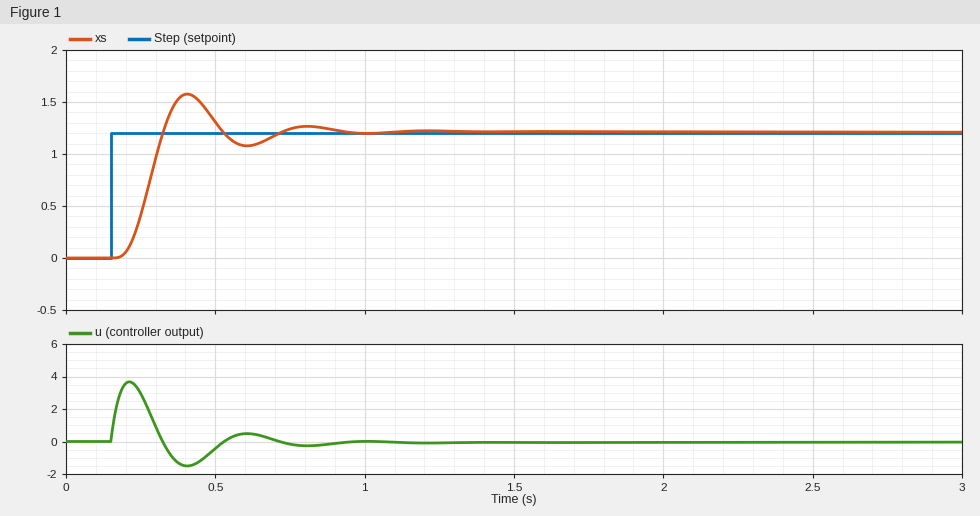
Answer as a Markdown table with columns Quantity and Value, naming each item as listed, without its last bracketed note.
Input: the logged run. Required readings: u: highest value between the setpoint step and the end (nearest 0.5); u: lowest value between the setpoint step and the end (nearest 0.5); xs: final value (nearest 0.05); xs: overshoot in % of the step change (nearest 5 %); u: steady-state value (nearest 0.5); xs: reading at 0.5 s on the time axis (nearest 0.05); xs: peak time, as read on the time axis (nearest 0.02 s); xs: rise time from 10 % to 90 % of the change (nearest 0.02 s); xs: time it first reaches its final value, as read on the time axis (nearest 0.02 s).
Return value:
| Quantity | Value |
|---|---|
| u: highest value between the setpoint step and the end | 3.5 |
| u: lowest value between the setpoint step and the end | -1.5 |
| xs: final value | 1.20 |
| xs: overshoot in % of the step change | 30 % |
| u: steady-state value | 0.0 |
| xs: reading at 0.5 s on the time axis | 1.30 |
| xs: peak time, as read on the time axis | 0.40 s |
| xs: rise time from 10 % to 90 % of the change | 0.10 s |
| xs: time it first reaches its final value, as read on the time axis | 0.32 s |
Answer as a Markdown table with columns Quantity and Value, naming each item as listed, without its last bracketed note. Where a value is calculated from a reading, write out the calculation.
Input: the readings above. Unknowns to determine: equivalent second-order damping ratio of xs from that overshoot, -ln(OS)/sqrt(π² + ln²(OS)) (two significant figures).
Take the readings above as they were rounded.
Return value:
| Quantity | Value |
|---|---|
| equivalent second-order damping ratio of xs from that overshoot, -ln(OS)/sqrt(π² + ln²(OS)) | ln(0.3) = -1.204; 1.204 / sqrt(9.870 + 1.450) = 0.36 |
